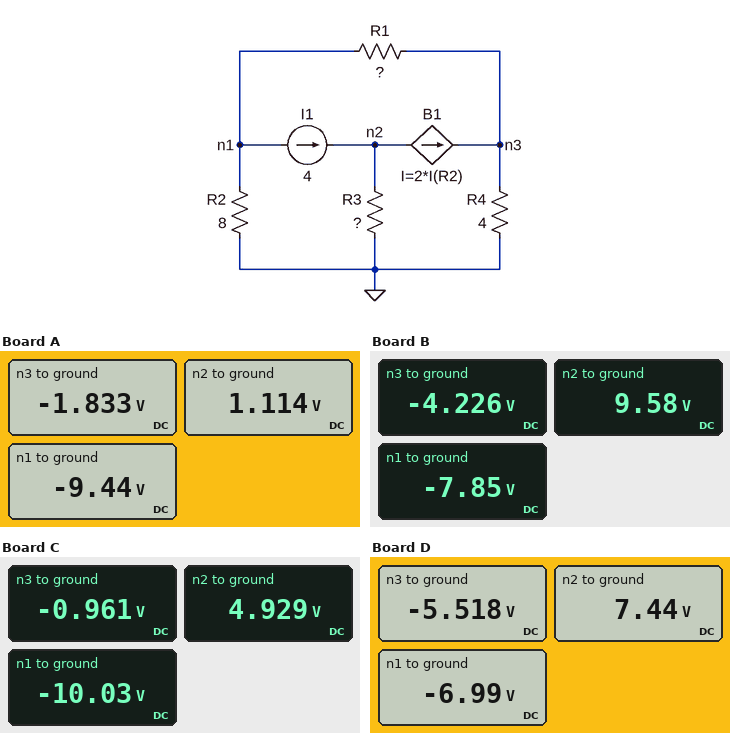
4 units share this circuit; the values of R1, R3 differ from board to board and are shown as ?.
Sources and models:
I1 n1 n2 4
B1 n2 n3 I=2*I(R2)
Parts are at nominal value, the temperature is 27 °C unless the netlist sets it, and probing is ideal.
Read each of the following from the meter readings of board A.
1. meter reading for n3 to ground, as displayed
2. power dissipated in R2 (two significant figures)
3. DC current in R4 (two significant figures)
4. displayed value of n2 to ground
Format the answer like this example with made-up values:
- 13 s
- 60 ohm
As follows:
- -1.833 V
- 11 W
- 460 mA
- 1.114 V
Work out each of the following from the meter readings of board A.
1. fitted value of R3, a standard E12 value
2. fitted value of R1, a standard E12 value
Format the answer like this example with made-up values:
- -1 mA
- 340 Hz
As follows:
- 0.68 Ω
- 2.7 Ω
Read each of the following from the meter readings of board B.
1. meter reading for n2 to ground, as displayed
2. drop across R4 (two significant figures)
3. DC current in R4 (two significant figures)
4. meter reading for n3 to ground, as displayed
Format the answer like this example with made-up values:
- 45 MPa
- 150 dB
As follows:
- 9.58 V
- 4.2 V
- 1.1 A
- -4.226 V
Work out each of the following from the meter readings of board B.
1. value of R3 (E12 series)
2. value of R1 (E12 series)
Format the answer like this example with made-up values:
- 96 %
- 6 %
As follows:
- 4.7 Ω
- 1.2 Ω
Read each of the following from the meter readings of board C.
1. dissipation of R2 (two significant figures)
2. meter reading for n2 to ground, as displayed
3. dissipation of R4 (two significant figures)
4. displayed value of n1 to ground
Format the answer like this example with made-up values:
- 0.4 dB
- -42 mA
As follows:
- 13 W
- 4.929 V
- 230 mW
- -10.03 V
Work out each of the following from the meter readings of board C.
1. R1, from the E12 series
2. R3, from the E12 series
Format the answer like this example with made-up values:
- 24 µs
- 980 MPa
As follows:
- 3.3 Ω
- 3.3 Ω
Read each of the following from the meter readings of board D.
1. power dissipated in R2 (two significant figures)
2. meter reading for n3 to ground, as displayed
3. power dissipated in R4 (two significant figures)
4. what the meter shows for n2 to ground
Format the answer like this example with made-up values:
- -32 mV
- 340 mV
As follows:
- 6.1 W
- -5.518 V
- 7.6 W
- 7.44 V
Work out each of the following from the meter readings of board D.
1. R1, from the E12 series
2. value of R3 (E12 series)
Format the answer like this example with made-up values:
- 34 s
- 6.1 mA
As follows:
- 0.47 Ω
- 3.3 Ω
